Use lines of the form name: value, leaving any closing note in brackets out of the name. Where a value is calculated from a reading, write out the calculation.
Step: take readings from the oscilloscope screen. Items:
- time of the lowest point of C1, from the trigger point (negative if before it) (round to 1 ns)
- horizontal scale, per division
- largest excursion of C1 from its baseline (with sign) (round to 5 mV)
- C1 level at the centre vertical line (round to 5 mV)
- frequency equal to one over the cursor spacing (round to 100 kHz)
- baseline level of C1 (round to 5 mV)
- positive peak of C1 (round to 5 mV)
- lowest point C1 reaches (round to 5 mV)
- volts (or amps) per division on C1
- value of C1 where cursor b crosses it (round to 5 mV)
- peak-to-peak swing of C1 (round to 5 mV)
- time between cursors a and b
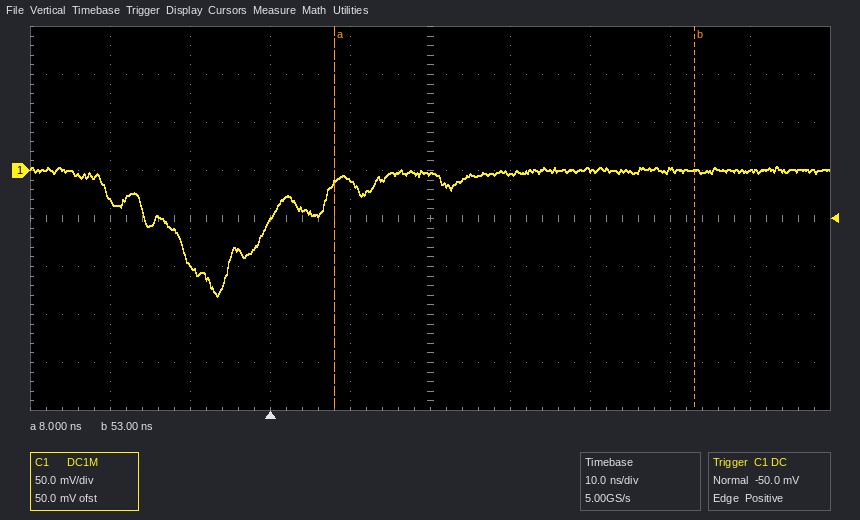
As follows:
time of the lowest point of C1, from the trigger point (negative if before it): -7 ns
horizontal scale, per division: 10 ns
largest excursion of C1 from its baseline (with sign): -130 mV − (0 mV) = -130 mV
C1 level at the centre vertical line: -5 mV
frequency equal to one over the cursor spacing: 1 / 45 ns ≈ 22.2 MHz
baseline level of C1: 0 mV
positive peak of C1: 5 mV
lowest point C1 reaches: -130 mV
volts (or amps) per division on C1: 50 mV
value of C1 where cursor b crosses it: 0 mV
peak-to-peak swing of C1: 5 mV − (-130 mV) = 135 mV
time between cursors a and b: 53 ns − (8 ns) = 45 ns
